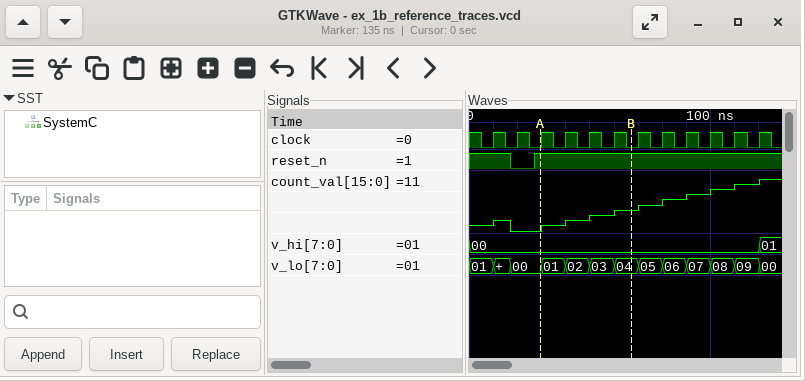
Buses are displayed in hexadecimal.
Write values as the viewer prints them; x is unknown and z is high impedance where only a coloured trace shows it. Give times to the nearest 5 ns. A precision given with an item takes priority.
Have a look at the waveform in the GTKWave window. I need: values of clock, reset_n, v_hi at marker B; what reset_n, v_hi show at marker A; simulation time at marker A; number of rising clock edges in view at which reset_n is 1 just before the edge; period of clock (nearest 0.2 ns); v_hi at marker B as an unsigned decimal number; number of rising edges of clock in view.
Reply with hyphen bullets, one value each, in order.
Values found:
- clock=0, reset_n=1, v_hi=00
- reset_n=1, v_hi=00
- 30 ns
- 11
- 10 ns
- 0
- 12
